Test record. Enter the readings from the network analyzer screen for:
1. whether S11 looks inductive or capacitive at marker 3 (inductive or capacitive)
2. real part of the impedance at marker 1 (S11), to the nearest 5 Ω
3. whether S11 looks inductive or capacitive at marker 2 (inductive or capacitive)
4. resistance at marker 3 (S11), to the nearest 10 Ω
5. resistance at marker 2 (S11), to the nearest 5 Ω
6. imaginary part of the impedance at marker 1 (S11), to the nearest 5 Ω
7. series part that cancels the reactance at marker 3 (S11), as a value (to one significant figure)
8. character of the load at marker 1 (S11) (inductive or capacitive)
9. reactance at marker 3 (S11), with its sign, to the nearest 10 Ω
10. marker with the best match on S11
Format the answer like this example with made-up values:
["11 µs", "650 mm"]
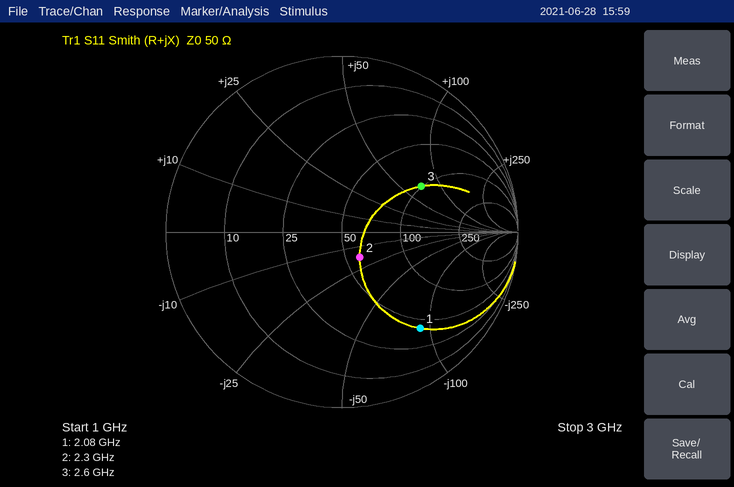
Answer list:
["inductive", "40 Ω", "capacitive", "100 Ω", "60 Ω", "-90 Ω", "900 fF", "capacitive", "+70 Ω", "marker 2"]
